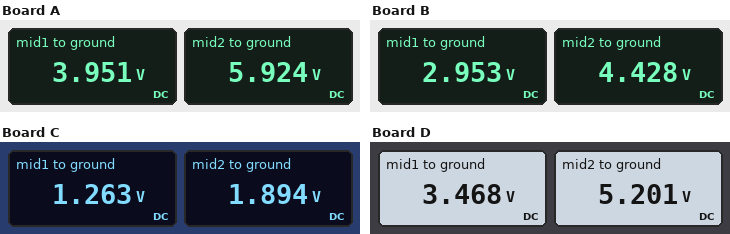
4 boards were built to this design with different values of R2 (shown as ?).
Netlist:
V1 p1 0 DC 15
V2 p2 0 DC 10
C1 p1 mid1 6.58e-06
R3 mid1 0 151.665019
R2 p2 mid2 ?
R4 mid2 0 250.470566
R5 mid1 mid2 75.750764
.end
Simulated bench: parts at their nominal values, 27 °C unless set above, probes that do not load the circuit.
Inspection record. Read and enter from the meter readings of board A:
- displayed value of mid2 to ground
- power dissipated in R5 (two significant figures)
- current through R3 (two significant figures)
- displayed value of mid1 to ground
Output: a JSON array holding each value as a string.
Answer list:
["5.924 V", "51 mW", "26 mA", "3.951 V"]
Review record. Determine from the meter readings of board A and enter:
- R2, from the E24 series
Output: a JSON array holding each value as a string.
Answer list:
["82 Ω"]
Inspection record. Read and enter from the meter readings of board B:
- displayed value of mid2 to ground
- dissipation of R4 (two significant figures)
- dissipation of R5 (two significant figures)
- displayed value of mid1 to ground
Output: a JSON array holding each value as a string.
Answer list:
["4.428 V", "78 mW", "29 mW", "2.953 V"]
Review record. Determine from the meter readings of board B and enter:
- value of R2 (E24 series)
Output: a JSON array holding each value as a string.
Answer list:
["150 Ω"]
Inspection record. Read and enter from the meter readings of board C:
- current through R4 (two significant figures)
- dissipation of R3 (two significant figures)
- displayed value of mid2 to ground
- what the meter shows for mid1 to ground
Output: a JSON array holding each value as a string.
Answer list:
["7.6 mA", "11 mW", "1.894 V", "1.263 V"]
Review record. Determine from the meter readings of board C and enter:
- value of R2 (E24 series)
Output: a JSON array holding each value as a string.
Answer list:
["510 Ω"]
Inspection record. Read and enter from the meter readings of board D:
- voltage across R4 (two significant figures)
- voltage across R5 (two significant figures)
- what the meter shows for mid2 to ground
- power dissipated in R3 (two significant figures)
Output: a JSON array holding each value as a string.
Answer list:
["5.2 V", "1.7 V", "5.201 V", "79 mW"]
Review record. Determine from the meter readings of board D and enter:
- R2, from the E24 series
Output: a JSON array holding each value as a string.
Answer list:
["110 Ω"]
